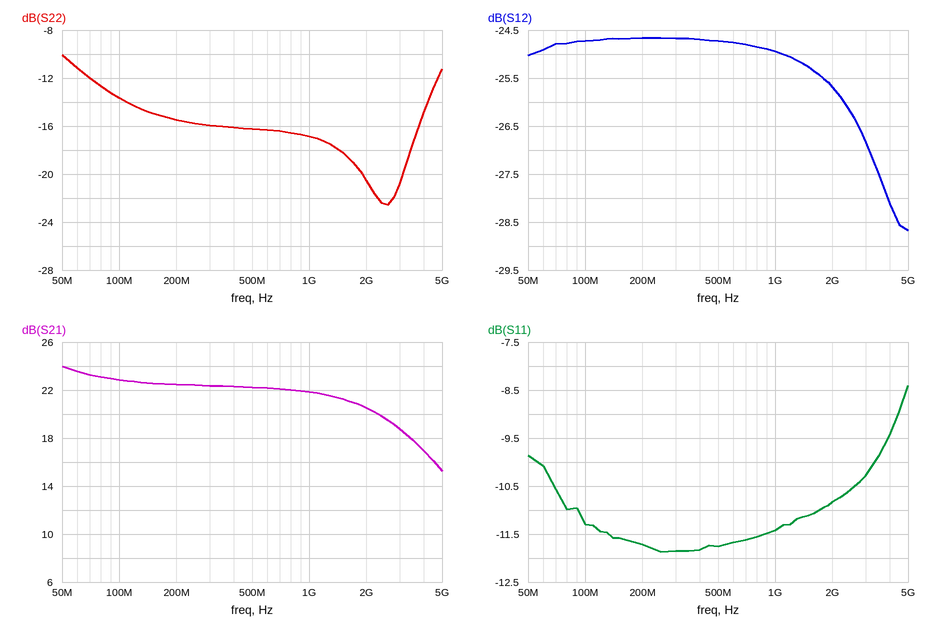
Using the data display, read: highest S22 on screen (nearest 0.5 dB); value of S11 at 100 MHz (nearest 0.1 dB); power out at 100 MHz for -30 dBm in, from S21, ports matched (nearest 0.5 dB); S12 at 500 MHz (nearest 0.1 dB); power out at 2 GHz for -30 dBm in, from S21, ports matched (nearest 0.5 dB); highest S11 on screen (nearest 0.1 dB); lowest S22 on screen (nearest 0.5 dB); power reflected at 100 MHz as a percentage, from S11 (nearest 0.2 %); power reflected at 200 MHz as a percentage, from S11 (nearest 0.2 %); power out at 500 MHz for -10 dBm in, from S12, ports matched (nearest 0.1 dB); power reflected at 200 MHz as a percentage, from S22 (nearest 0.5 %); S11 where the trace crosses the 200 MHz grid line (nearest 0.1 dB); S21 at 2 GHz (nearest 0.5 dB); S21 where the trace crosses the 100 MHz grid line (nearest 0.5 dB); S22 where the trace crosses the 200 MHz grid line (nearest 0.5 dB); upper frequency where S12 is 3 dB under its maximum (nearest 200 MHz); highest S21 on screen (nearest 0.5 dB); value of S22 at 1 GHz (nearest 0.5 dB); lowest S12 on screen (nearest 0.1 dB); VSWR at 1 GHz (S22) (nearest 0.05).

-10.0 dB
-11.3 dB
-7.0 dBm
-24.7 dB
-9.5 dBm
-8.4 dB
-22.5 dB
7.4 %
6.8 %
-34.7 dBm
3.0 %
-11.7 dB
20.5 dB
23.0 dB
-15.5 dB
3.6 GHz
24.0 dB
-17.0 dB
-28.7 dB
1.35
